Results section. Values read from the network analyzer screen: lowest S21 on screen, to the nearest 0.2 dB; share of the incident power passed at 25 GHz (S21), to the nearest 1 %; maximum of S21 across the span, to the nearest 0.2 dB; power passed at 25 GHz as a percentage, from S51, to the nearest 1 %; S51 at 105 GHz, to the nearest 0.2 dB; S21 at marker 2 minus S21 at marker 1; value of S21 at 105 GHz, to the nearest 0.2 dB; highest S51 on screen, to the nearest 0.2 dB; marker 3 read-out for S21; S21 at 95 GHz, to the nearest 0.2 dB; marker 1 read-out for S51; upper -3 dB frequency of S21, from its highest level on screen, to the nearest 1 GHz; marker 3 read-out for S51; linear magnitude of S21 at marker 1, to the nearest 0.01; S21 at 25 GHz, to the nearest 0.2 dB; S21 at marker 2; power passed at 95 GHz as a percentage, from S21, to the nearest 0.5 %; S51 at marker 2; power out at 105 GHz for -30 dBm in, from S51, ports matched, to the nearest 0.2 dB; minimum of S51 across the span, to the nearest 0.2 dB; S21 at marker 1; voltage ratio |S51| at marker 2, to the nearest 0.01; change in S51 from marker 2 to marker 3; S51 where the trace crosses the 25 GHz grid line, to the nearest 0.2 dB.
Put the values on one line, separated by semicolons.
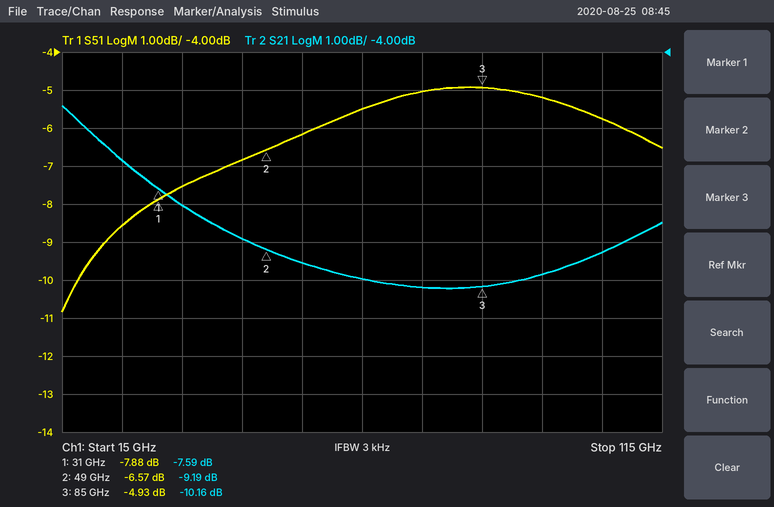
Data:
-10.2 dB; 21 %; -5.4 dB; 14 %; -5.8 dB; -1.60 dB; -9.2 dB; -5.0 dB; -10.16 dB; -9.8 dB; -7.88 dB; 39 GHz; -4.93 dB; 0.42; -6.8 dB; -9.19 dB; 10.5 %; -6.57 dB; -35.8 dBm; -10.8 dB; -7.59 dB; 0.47; 1.64 dB; -8.6 dB
